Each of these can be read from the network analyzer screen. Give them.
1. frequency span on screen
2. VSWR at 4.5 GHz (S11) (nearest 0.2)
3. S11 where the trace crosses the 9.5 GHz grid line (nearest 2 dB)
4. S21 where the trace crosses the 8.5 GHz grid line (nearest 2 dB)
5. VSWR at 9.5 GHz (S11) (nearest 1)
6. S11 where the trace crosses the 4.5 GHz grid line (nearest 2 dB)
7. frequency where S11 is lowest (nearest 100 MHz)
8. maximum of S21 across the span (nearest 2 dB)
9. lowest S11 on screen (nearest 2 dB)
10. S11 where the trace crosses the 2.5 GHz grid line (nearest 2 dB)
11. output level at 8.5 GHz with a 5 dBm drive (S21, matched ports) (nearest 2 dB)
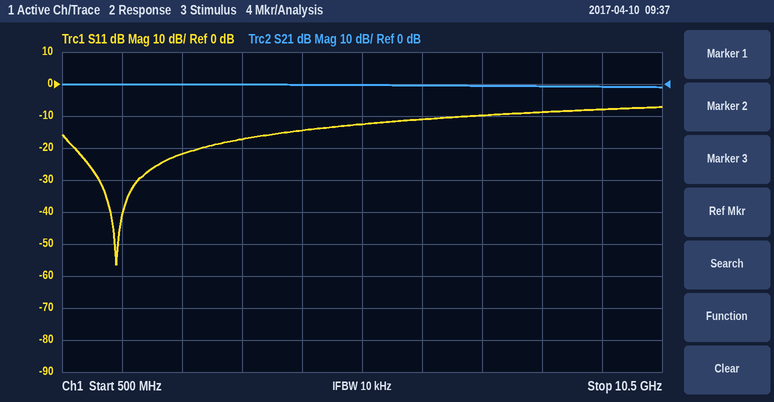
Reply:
10 GHz
1.4
-8 dB
0 dB
2
-14 dB
1.4 GHz
0 dB
-56 dB
-22 dB
4 dBm
